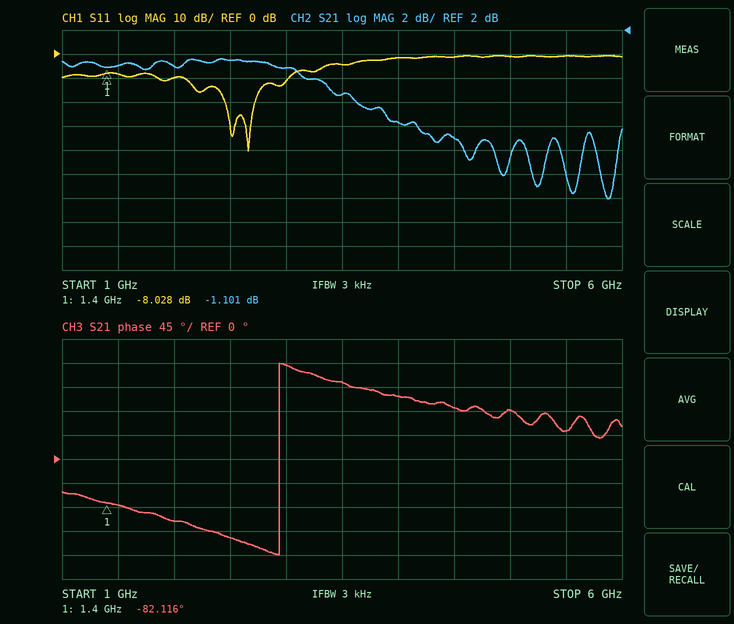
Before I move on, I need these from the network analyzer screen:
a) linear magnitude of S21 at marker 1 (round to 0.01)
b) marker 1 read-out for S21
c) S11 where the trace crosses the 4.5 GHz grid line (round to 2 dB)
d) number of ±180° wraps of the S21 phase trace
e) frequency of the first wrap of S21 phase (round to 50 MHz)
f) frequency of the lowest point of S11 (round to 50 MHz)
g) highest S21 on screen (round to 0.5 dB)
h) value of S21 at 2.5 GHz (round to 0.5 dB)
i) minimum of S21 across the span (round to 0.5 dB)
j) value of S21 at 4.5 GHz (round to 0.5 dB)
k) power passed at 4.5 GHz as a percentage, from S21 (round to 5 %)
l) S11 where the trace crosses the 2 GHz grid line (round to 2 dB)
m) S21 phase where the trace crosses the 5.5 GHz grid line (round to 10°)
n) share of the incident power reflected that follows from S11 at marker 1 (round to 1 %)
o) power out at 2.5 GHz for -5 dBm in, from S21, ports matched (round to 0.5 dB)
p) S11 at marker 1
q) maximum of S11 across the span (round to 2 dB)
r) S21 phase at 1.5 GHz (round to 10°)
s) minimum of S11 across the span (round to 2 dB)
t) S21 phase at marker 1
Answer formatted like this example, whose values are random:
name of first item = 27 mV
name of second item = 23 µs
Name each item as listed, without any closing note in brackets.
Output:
linear magnitude of S21 at marker 1 = 0.88
marker 1 read-out for S21 = -1.101 dB
S11 where the trace crosses the 4.5 GHz grid line = -2 dB
number of ±180° wraps of the S21 phase trace = 1
frequency of the first wrap of S21 phase = 2.95 GHz
frequency of the lowest point of S11 = 2.65 GHz
highest S21 on screen = -0.5 dB
value of S21 at 2.5 GHz = -0.5 dB
minimum of S21 across the span = -12.0 dB
value of S21 at 4.5 GHz = -7.0 dB
power passed at 4.5 GHz as a percentage, from S21 = 20 %
S11 where the trace crosses the 2 GHz grid line = -10 dB
S21 phase where the trace crosses the 5.5 GHz grid line = 50°
share of the incident power reflected that follows from S11 at marker 1 = 16 %
power out at 2.5 GHz for -5 dBm in, from S21, ports matched = -5.5 dBm
S11 at marker 1 = -8.028 dB
maximum of S11 across the span = 0 dB
S21 phase at 1.5 GHz = -90°
minimum of S11 across the span = -40 dB
S21 phase at marker 1 = -82.116°
